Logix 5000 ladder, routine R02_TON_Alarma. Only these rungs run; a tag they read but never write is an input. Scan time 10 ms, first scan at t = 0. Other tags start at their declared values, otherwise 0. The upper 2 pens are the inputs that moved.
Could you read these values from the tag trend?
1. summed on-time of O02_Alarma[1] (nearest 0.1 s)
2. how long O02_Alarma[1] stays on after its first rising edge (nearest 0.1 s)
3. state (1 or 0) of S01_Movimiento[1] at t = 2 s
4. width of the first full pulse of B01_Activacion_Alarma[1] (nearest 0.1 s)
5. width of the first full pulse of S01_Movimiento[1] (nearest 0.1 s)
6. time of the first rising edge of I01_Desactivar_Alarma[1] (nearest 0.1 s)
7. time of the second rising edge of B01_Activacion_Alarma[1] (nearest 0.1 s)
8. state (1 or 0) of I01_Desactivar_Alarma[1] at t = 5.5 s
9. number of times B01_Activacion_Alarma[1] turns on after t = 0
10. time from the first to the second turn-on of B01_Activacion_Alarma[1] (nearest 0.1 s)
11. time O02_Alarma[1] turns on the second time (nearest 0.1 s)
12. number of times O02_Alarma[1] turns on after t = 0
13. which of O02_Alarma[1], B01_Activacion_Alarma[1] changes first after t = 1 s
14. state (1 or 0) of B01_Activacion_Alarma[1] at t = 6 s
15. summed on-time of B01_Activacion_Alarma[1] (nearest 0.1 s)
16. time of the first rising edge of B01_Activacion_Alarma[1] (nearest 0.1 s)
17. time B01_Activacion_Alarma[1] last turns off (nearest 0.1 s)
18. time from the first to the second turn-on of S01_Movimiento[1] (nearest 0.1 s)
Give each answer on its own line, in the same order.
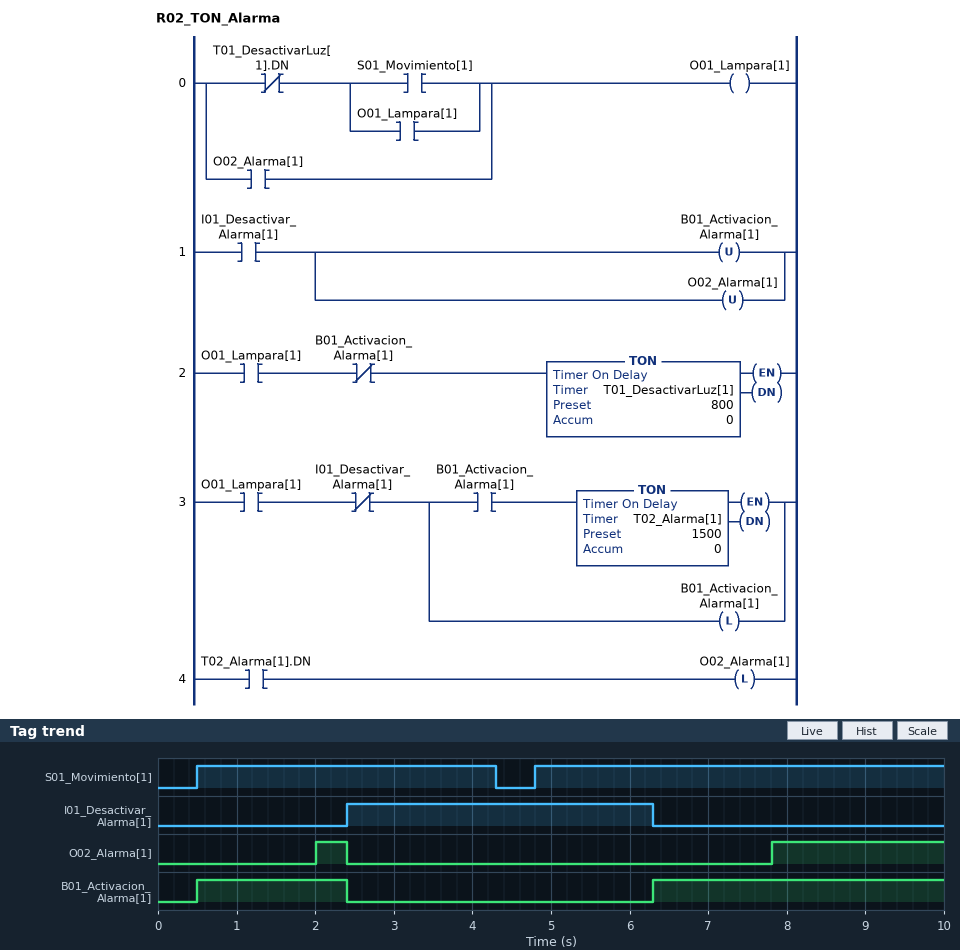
2.6 s
0.4 s
1
1.9 s
3.8 s
2.4 s
6.3 s
1
2
5.8 s
7.8 s
2
O02_Alarma[1]
0
5.6 s
0.5 s
2.4 s
4.3 s
